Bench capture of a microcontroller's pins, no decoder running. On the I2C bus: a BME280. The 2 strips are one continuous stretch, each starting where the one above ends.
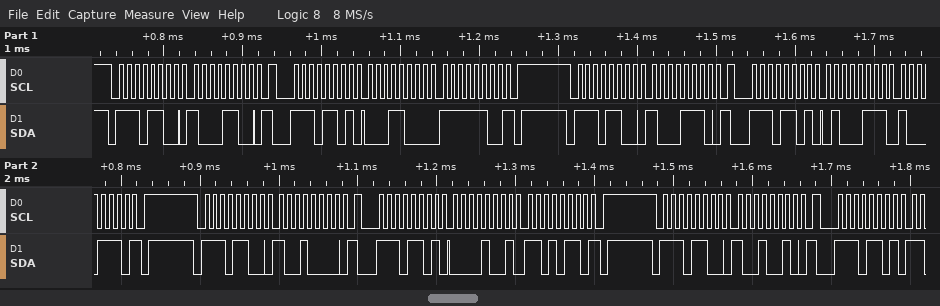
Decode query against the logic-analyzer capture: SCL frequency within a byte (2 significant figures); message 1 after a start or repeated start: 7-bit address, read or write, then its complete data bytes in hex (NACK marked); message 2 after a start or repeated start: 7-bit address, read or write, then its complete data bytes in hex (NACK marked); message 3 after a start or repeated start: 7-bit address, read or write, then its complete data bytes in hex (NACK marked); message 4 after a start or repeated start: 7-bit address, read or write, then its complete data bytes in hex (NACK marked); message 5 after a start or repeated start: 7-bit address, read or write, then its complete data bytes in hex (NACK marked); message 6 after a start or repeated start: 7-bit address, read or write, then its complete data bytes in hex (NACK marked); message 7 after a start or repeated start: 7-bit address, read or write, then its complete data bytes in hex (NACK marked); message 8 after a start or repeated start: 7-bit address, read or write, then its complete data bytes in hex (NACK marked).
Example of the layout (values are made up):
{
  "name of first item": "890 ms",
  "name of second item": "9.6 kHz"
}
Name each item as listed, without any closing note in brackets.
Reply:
{
  "SCL frequency within a byte": "100 kHz",
  "message 1 after a start or repeated start: 7-bit address, read or write, then its complete data bytes in hex": "0x76 write: 8C",
  "message 2 after a start or repeated start: 7-bit address, read or write, then its complete data bytes in hex": "0x76 read: 18 FC NACK",
  "message 3 after a start or repeated start: 7-bit address, read or write, then its complete data bytes in hex": "0x76 write: 8E",
  "message 4 after a start or repeated start: 7-bit address, read or write, then its complete data bytes in hex": "0x76 read: 47 8E NACK",
  "message 5 after a start or repeated start: 7-bit address, read or write, then its complete data bytes in hex": "0x76 write: 90",
  "message 6 after a start or repeated start: 7-bit address, read or write, then its complete data bytes in hex": "0x76 read: 09 D6 NACK",
  "message 7 after a start or repeated start: 7-bit address, read or write, then its complete data bytes in hex": "0x76 write: 92",
  "message 8 after a start or repeated start: 7-bit address, read or write, then its complete data bytes in hex": "0x76 read"
}
